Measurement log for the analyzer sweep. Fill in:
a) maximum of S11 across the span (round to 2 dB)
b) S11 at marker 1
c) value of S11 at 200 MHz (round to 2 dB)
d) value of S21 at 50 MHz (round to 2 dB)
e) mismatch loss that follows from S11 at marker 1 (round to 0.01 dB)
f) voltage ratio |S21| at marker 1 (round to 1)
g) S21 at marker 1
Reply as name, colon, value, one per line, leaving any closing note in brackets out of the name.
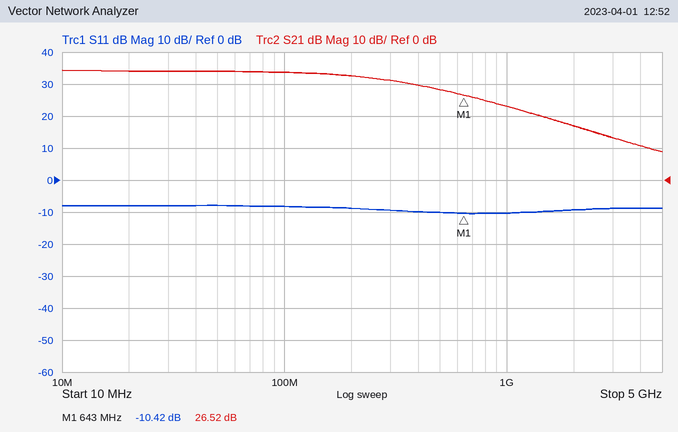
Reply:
maximum of S11 across the span: -8 dB
S11 at marker 1: -10.42 dB
value of S11 at 200 MHz: -8 dB
value of S21 at 50 MHz: 34 dB
mismatch loss that follows from S11 at marker 1: 0.41 dB
voltage ratio |S21| at marker 1: 21
S21 at marker 1: 26.52 dB
